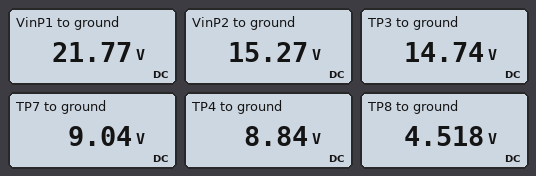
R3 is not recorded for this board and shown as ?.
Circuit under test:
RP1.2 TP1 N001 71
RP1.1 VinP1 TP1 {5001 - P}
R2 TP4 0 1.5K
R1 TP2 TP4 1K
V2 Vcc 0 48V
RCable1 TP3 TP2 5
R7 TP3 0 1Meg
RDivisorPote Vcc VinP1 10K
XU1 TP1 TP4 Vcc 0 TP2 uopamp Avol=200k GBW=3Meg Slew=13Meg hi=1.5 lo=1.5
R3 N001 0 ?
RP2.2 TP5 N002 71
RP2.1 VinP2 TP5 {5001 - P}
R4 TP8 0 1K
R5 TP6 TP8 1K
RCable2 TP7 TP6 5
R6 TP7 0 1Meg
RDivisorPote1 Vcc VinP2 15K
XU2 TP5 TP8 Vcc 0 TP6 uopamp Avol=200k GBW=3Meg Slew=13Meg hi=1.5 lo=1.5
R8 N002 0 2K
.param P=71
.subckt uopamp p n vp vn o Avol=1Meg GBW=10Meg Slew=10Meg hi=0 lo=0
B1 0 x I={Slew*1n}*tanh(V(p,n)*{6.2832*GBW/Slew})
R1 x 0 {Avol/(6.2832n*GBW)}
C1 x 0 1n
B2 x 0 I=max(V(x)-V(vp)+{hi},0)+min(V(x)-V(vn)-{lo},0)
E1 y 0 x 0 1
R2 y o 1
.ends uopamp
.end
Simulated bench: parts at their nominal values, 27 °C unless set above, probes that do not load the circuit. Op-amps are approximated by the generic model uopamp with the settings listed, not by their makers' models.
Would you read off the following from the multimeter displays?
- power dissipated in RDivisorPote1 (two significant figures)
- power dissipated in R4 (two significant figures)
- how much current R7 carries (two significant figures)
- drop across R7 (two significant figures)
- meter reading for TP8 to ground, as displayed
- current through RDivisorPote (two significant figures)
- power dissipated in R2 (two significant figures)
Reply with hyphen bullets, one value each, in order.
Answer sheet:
- 71 mW
- 20 mW
- 15 µA
- 15 V
- 4.518 V
- 2.6 mA
- 52 mW
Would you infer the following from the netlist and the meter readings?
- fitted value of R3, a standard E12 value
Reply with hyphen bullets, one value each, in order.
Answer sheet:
- 3.3 kΩ
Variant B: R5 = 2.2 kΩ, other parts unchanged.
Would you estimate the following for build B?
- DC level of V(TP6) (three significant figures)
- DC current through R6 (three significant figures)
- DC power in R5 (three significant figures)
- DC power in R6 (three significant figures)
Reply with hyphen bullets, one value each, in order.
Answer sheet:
- 14.5 V
- 14.5 µA
- 44.9 mW
- 209 µW
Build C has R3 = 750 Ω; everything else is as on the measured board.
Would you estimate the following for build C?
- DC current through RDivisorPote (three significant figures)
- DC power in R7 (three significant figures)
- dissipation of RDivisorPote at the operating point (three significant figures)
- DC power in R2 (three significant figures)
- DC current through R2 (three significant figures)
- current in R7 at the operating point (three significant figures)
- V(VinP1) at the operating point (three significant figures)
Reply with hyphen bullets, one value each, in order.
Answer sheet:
- 3.05 mA
- 17.4 µW
- 92.9 mW
- 4.17 mW
- 1.67 mA
- 4.17 µA
- 17.5 V
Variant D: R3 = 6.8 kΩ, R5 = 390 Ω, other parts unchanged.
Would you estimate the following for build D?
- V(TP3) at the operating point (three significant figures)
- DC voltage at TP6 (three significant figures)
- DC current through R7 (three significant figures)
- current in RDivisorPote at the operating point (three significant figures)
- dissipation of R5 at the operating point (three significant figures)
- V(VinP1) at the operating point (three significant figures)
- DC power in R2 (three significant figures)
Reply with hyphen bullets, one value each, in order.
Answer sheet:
- 25.2 V
- 6.28 V
- 25.2 µA
- 2.20 mA
- 7.96 mW
- 26.0 V
- 153 mW
